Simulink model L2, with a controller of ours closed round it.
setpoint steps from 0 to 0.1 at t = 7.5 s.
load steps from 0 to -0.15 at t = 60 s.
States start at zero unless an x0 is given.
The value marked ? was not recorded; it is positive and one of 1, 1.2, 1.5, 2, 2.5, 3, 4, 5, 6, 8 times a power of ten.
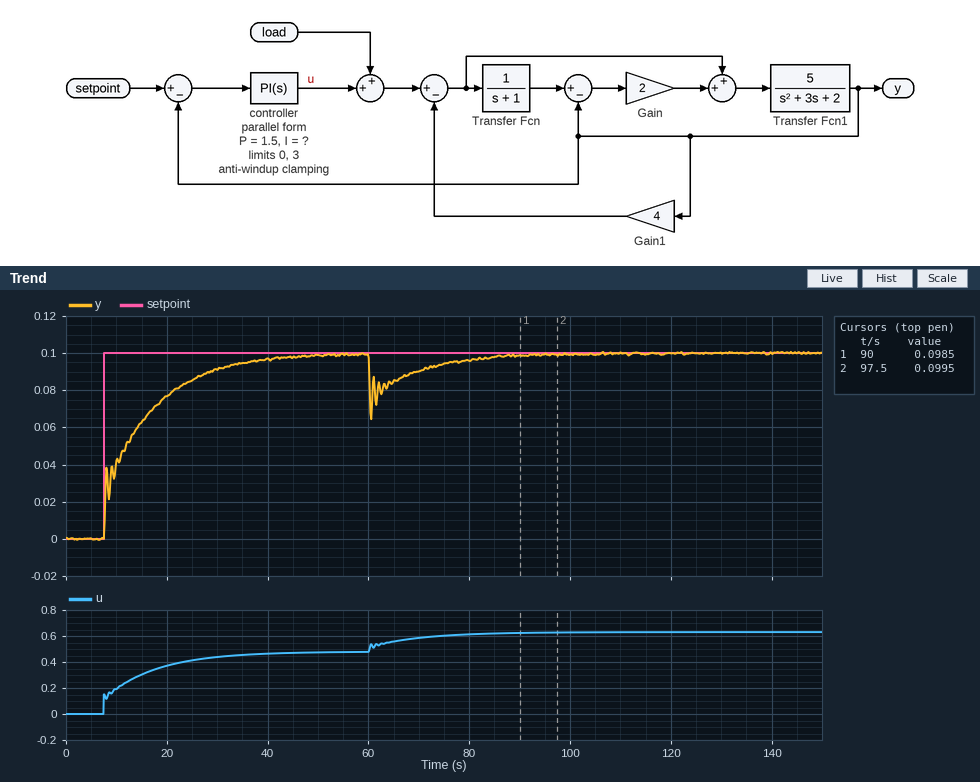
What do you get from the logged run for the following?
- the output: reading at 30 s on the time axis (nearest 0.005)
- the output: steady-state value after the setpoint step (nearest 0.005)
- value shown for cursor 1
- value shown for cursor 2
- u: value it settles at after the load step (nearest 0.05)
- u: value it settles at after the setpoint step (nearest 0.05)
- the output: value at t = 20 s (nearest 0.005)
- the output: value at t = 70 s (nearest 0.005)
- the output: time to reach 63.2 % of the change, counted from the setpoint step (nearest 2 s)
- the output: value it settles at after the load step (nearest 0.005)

0.090
0.100
0.0985
0.0995
0.65
0.50
0.075
0.090
8 s
0.100
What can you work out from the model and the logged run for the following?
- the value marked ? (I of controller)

0.6
